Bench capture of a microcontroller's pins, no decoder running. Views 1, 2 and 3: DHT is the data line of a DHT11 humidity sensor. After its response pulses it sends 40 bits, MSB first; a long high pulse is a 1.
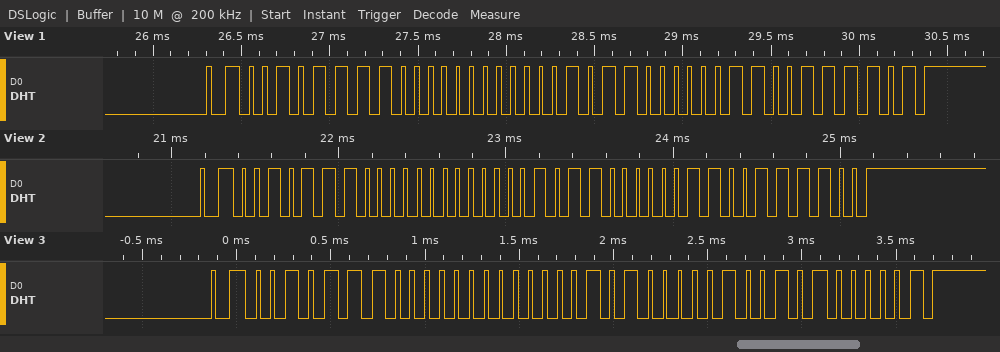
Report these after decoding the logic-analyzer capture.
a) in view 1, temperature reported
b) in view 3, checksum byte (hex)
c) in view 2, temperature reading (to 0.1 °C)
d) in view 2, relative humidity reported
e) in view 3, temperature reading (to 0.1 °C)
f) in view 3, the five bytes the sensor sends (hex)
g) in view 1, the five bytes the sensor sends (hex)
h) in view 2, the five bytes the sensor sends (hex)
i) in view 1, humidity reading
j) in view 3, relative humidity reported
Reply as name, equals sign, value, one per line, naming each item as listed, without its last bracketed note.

in view 1, temperature reported = 11.3 °C
in view 3, checksum byte = 0x41
in view 2, temperature reading = 11.3 °C
in view 2, relative humidity reported = 46 %
in view 3, temperature reading = 10.9 °C
in view 3, the five bytes the sensor sends = 2E 00 0A 09 41
in view 1, the five bytes the sensor sends = 2F 00 0B 03 3D
in view 2, the five bytes the sensor sends = 2E 00 0B 03 3C
in view 1, humidity reading = 47 %
in view 3, relative humidity reported = 46 %
